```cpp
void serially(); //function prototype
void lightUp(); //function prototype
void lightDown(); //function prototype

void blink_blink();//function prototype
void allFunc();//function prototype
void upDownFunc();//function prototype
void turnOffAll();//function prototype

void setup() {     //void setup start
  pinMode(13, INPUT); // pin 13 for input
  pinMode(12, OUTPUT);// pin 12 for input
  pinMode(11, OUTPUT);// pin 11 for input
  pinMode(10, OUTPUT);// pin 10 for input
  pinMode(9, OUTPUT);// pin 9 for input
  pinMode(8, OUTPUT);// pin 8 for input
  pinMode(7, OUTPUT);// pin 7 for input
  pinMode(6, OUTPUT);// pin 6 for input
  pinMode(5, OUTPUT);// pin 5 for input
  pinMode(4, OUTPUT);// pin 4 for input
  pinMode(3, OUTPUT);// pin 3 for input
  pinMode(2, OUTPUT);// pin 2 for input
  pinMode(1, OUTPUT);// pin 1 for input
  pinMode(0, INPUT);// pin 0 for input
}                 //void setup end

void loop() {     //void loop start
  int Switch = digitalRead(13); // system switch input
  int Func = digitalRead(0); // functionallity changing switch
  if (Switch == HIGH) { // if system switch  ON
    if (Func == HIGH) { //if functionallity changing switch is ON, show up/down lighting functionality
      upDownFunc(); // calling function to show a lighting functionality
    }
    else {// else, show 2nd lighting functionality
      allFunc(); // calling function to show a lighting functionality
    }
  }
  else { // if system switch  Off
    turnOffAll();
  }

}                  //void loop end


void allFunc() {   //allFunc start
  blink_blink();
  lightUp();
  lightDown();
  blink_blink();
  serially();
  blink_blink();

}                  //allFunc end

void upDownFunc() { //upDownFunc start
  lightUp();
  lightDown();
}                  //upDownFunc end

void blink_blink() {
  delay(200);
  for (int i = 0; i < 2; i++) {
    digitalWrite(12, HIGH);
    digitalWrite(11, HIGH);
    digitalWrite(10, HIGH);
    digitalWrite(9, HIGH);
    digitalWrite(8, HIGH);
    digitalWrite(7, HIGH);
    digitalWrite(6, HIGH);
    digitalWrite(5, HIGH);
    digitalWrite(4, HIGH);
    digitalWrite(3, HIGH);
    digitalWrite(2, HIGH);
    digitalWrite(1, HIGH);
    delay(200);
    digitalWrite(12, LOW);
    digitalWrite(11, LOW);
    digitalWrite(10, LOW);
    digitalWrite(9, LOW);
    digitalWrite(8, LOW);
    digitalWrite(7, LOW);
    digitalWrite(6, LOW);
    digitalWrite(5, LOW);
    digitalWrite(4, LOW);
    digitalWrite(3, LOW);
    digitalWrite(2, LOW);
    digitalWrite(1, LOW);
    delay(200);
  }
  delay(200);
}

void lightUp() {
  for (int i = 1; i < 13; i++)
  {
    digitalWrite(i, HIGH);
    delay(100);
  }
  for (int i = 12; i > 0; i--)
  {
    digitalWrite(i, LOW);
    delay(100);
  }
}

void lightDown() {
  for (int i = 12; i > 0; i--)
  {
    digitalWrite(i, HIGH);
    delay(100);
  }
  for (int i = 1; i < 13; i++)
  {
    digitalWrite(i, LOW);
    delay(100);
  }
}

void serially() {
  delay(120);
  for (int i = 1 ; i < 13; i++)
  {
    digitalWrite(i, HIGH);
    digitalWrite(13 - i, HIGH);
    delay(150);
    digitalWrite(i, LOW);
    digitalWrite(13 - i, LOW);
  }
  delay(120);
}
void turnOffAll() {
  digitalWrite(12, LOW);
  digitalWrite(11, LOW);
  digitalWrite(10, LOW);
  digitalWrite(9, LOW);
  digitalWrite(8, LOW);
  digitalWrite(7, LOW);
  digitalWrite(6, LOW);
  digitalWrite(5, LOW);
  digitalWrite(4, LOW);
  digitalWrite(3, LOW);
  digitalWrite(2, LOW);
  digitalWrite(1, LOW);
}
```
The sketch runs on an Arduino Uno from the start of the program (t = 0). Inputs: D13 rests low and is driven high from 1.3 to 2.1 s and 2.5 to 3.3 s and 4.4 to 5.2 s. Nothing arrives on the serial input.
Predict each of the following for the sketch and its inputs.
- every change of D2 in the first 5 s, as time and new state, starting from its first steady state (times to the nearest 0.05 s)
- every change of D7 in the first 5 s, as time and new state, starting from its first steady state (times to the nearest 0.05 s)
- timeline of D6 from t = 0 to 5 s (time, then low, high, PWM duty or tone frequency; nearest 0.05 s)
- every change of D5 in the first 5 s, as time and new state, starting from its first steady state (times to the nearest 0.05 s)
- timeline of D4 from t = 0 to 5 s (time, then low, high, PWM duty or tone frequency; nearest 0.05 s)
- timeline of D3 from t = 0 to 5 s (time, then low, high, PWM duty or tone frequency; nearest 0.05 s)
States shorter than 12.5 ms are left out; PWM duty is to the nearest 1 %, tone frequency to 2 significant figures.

0 s low; 1.5 s high; 1.7 s low; 1.9 s high; 2.1 s low; 2.6 s high; 4.7 s low
0 s low; 1.5 s high; 1.7 s low; 1.9 s high; 2.1 s low; 3.1 s high; 4.2 s low
0 s low; 1.5 s high; 1.7 s low; 1.9 s high; 2.1 s low; 3 s high; 4.3 s low
0 s low; 1.5 s high; 1.7 s low; 1.9 s high; 2.1 s low; 2.9 s high; 4.4 s low
0 s low; 1.5 s high; 1.7 s low; 1.9 s high; 2.1 s low; 2.8 s high; 4.5 s low
0 s low; 1.5 s high; 1.7 s low; 1.9 s high; 2.1 s low; 2.7 s high; 4.6 s low
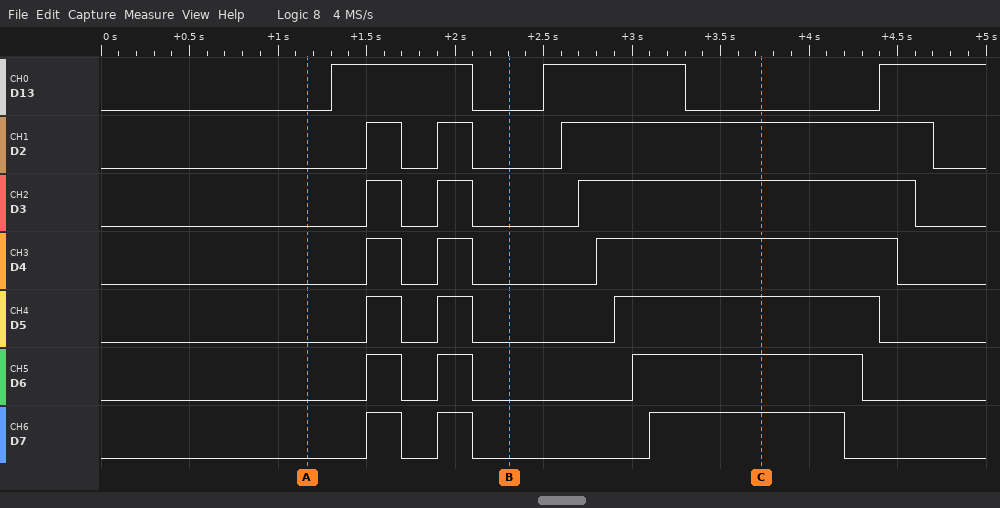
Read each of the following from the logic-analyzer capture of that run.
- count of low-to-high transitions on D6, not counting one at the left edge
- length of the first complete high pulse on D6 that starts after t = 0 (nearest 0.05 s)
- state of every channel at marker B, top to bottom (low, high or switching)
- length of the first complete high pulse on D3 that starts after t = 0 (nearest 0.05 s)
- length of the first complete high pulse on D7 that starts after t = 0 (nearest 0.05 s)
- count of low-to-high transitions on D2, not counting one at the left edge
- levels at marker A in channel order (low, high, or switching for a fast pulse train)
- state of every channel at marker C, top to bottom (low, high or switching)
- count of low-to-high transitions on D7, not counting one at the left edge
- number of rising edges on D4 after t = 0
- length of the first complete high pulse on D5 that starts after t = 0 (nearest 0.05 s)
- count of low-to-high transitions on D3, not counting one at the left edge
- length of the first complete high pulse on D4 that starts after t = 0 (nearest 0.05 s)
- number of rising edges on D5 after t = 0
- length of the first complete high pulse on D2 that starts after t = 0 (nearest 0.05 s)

3
0.20 s
D13 low, D2 low, D3 low, D4 low, D5 low, D6 low, D7 low
0.20 s
0.20 s
3
D13 low, D2 low, D3 low, D4 low, D5 low, D6 low, D7 low
D13 low, D2 high, D3 high, D4 high, D5 high, D6 high, D7 high
3
3
0.20 s
3
0.20 s
3
0.20 s
